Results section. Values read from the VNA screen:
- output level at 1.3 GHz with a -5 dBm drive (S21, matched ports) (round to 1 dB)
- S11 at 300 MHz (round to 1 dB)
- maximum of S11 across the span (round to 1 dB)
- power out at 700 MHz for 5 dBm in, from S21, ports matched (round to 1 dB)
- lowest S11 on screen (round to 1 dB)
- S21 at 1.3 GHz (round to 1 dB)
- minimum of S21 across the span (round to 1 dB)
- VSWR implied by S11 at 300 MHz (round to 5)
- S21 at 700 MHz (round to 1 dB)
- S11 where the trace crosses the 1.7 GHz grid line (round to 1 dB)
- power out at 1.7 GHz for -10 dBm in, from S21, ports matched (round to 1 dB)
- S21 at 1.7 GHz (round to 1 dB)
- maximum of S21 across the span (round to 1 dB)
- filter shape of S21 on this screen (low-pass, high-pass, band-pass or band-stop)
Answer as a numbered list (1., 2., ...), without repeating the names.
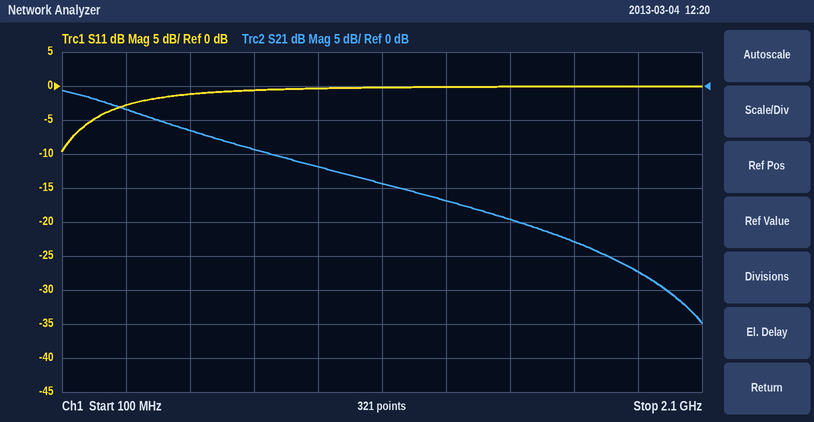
1. -22 dBm
2. -3 dB
3. 0 dB
4. -4 dBm
5. -10 dB
6. -17 dB
7. -35 dB
8. 5
9. -9 dB
10. 0 dB
11. -33 dBm
12. -23 dB
13. -1 dB
14. low-pass
